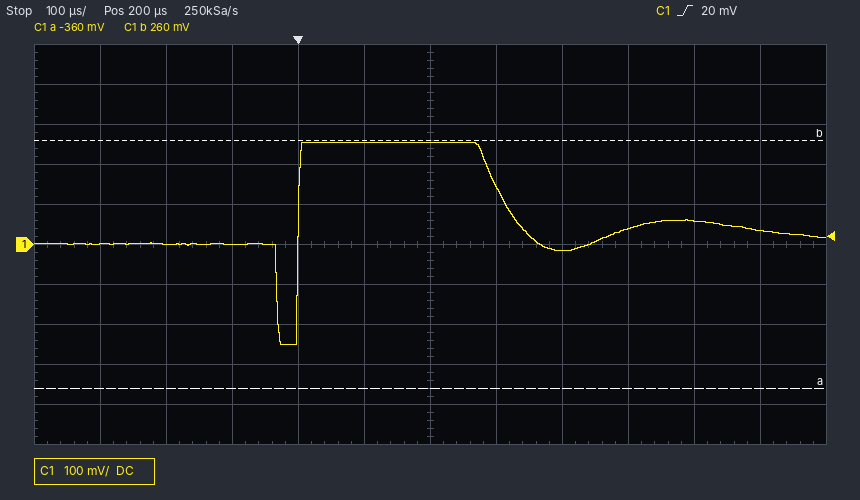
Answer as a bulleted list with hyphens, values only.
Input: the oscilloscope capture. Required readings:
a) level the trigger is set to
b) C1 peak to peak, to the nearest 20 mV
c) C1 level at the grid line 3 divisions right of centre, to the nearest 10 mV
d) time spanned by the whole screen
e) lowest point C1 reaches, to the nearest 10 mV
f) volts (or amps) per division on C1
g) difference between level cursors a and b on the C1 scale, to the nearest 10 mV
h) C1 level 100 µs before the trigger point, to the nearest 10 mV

- 20 mV
- 500 mV
- 40 mV
- 1.2 ms
- -250 mV
- 100 mV
- 620 mV
- 0 mV
